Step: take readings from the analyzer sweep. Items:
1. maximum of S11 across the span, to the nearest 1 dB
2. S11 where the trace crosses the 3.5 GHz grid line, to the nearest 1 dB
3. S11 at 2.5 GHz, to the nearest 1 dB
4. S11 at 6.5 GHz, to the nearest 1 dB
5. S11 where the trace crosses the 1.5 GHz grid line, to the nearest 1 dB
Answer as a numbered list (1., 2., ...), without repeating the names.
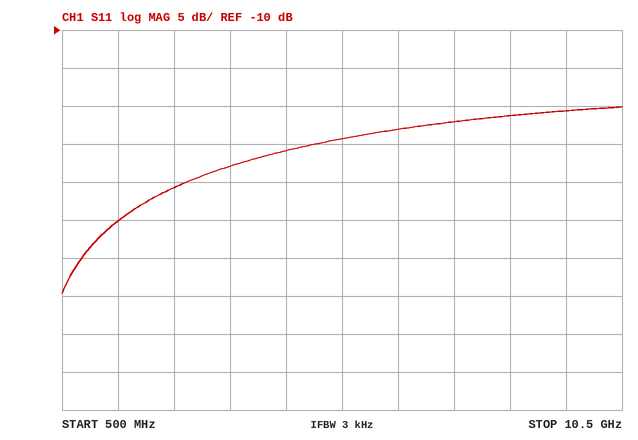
1. -20 dB
2. -28 dB
3. -31 dB
4. -23 dB
5. -35 dB
